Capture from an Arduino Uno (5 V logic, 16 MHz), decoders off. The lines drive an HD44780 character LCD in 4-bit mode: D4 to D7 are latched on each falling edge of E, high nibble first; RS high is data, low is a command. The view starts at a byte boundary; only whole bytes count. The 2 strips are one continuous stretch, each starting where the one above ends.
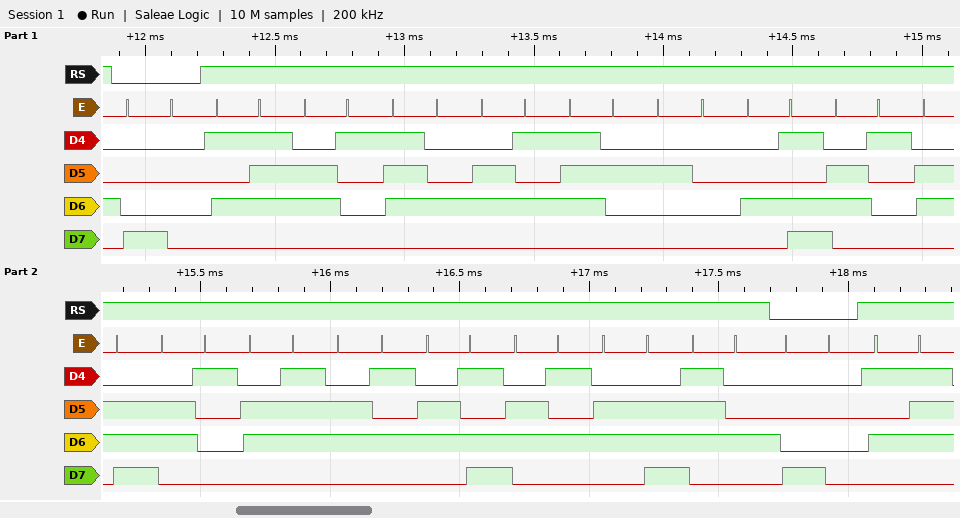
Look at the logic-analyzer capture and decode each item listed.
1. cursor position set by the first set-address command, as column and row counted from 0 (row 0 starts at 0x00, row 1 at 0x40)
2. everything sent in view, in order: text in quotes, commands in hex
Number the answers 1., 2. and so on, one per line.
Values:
1. column 0, row 0
2. 0x80 "Water Management" 0x80 "W"
